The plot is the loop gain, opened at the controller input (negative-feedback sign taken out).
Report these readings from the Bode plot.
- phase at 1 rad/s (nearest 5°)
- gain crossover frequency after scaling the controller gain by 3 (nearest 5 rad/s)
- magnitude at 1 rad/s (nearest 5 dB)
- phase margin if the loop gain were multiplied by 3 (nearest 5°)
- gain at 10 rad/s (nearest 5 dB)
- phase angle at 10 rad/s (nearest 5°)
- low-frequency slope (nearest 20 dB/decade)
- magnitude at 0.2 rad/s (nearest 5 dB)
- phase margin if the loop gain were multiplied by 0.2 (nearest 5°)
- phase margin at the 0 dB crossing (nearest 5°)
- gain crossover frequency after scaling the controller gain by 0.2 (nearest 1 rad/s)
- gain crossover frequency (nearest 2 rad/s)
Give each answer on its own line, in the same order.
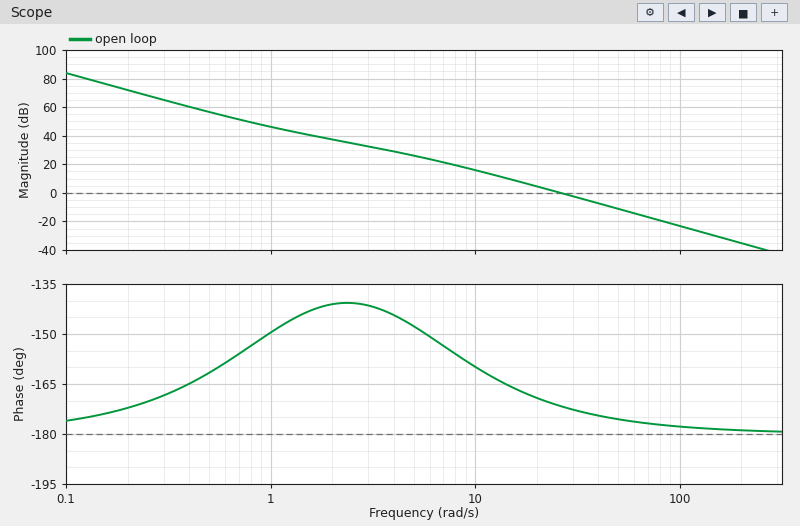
-150°
45 rad/s
45 dB
5°
15 dB
-160°
-40 dB/decade
70 dB
20°
10°
11 rad/s
26 rad/s
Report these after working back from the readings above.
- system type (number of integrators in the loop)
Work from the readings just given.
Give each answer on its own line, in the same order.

2
